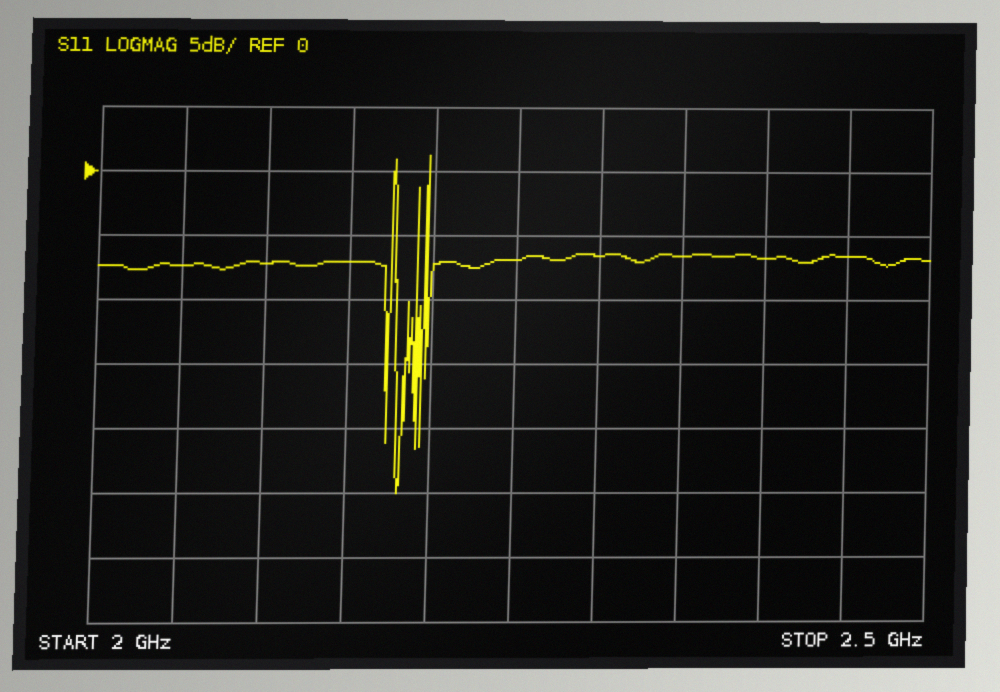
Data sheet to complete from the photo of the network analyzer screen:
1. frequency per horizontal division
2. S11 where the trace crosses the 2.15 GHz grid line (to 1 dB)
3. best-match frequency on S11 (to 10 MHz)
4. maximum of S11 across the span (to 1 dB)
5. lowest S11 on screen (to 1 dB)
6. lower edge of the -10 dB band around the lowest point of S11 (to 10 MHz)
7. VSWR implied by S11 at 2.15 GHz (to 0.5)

50 MHz
-7 dB
2.18 GHz
1 dB
-25 dB
2.18 GHz
2.5
